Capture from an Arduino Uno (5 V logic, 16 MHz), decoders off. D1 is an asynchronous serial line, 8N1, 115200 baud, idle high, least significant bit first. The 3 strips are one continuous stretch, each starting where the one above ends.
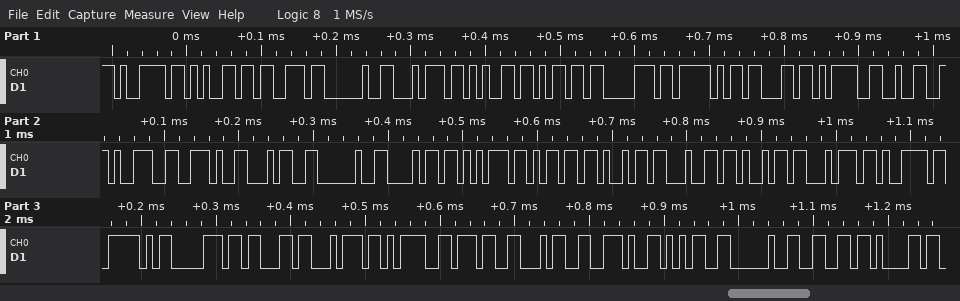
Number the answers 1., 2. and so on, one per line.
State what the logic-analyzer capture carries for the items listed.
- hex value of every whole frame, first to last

1. 79 65 73 20 74 65 6D 70 5F 63 3D 32 39 2E 34 20 68 75 6D 69 64 69 74 79 5F 70 63 74 3D 37 34 2E 35 20 66 61
